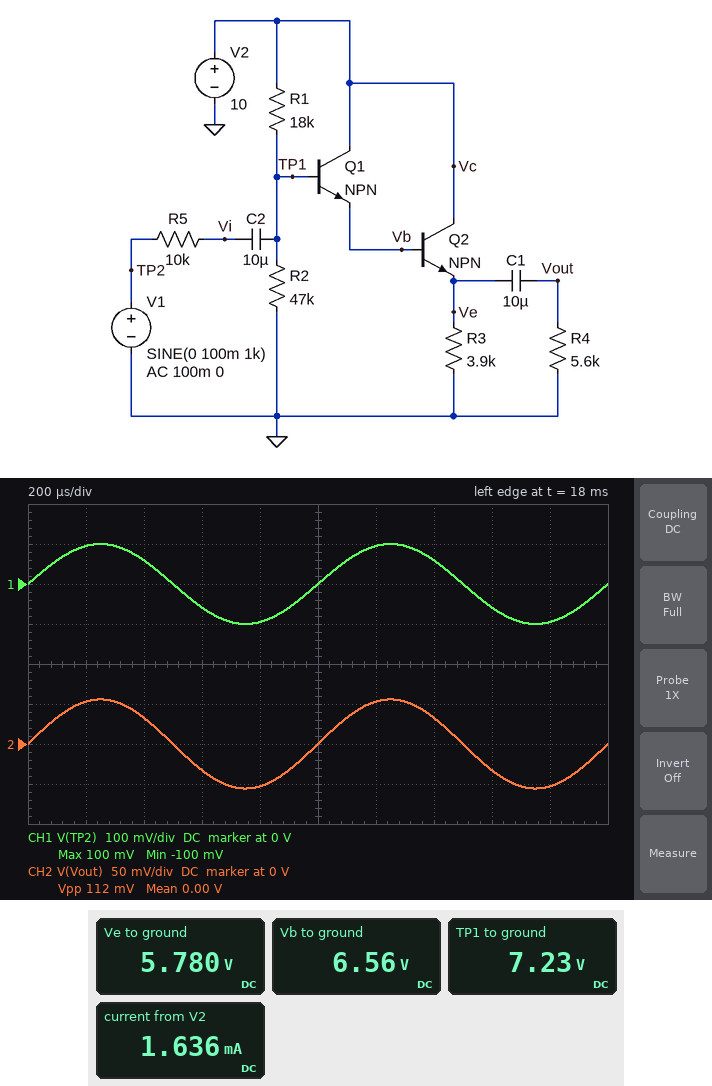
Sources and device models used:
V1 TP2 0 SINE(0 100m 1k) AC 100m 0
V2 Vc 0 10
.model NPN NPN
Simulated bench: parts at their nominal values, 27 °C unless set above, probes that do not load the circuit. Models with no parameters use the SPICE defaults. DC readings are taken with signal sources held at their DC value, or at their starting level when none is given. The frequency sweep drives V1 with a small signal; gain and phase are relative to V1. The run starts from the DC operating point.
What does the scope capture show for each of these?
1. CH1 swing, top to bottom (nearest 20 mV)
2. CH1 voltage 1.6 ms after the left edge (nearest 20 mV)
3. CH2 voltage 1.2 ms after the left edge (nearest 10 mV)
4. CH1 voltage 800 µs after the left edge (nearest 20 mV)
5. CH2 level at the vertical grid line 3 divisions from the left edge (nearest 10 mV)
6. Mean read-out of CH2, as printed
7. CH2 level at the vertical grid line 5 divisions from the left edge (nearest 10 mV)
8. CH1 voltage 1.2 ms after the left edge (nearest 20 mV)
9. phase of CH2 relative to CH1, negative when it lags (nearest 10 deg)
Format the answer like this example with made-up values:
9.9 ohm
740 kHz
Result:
200 mV
-60 mV
50 mV
-100 mV
-30 mV
0.00 V
0 V
100 mV
0 deg
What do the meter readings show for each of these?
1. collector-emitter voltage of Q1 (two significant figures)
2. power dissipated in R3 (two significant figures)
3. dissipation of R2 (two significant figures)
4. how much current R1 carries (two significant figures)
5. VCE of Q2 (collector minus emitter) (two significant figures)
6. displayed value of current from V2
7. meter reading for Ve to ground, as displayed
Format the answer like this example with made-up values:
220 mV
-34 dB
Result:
3.4 V
8.6 mW
1.1 mW
150 µA
4.2 V
1.636 mA
5.780 V
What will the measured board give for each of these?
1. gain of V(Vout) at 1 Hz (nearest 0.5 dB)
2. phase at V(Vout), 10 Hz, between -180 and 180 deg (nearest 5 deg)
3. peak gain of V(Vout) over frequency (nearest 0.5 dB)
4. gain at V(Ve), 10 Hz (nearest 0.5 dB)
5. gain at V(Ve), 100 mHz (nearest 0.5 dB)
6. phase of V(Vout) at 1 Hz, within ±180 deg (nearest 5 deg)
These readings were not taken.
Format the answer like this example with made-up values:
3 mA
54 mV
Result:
-16.5 dB
20 deg
-5.0 dB
-5.0 dB
-22.0 dB
105 deg
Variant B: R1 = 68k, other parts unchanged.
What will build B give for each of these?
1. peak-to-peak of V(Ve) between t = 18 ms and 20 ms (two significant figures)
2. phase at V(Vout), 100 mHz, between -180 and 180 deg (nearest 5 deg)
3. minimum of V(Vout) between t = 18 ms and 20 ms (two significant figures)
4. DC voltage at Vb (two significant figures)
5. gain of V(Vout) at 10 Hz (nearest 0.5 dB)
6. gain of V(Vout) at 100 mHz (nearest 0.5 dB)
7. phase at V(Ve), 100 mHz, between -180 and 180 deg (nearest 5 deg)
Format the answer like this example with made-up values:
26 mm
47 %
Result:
140 mV
165 deg
-71 mV
3.4 V
-3.5 dB
-44.5 dB
75 deg
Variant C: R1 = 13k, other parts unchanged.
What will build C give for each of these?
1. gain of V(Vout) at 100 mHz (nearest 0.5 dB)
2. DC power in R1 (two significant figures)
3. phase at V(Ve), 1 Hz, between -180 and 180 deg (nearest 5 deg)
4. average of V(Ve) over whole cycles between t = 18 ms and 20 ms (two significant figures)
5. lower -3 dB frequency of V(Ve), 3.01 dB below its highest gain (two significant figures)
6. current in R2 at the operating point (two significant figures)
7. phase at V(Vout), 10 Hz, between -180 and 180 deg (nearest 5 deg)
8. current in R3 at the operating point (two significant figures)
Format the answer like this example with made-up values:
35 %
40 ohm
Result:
-53.0 dB
360 µW
40 deg
6.4 V
780 mHz
170 µA
20 deg
1.6 mA
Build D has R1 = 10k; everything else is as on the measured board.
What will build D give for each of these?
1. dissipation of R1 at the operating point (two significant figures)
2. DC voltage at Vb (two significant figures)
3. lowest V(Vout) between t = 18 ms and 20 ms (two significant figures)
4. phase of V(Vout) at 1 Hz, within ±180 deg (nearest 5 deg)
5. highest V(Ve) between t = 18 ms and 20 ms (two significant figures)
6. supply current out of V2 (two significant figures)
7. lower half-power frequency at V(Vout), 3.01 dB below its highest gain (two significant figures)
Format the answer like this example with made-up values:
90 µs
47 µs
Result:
310 µW
7.6 V
-45 mV
110 deg
6.8 V
1.9 mA
3.1 Hz
